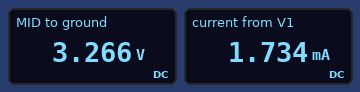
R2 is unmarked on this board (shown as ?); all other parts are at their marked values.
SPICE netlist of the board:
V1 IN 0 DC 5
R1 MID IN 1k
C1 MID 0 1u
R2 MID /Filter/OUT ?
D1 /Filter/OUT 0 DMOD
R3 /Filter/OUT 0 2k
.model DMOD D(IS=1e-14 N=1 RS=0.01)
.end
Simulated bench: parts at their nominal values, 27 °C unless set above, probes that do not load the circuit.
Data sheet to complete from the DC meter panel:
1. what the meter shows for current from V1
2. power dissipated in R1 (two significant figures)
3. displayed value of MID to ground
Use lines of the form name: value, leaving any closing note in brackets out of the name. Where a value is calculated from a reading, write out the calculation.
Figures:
what the meter shows for current from V1: 1.734 mA
power dissipated in R1: (5 V - 3.266 V)^2 / 1 kΩ = 3.0 mW
displayed value of MID to ground: 3.266 V
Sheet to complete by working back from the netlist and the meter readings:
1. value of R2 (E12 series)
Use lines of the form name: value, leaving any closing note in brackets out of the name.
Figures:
value of R2: 1.5 kΩ
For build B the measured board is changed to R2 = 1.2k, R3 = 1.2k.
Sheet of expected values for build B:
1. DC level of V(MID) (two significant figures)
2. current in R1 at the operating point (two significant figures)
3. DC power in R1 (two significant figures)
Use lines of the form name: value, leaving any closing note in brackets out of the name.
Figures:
DC level of V(MID): 3.0 V
current in R1 at the operating point: 2.0 mA
DC power in R1: 3.9 mW
